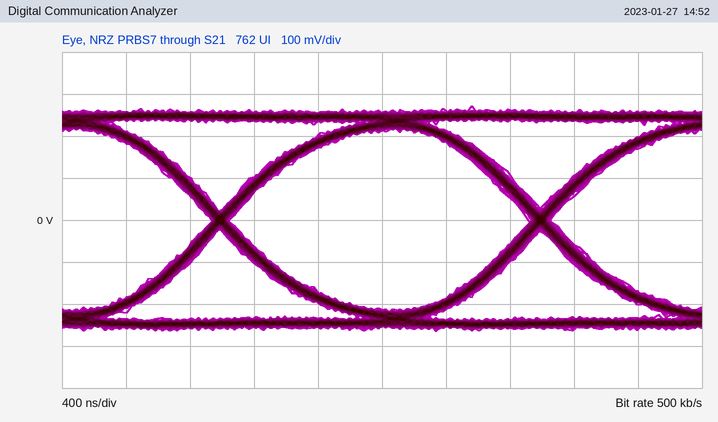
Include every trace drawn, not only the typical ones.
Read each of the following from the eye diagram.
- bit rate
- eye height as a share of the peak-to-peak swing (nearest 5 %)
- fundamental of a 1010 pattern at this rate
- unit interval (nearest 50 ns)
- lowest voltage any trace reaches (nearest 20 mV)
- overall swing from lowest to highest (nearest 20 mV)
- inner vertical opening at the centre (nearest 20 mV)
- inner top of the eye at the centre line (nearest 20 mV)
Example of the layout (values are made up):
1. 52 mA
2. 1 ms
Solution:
1. 500 kb/s
2. 80 %
3. 250 kHz
4. 2.00 µs
5. -260 mV
6. 540 mV
7. 420 mV
8. 220 mV
